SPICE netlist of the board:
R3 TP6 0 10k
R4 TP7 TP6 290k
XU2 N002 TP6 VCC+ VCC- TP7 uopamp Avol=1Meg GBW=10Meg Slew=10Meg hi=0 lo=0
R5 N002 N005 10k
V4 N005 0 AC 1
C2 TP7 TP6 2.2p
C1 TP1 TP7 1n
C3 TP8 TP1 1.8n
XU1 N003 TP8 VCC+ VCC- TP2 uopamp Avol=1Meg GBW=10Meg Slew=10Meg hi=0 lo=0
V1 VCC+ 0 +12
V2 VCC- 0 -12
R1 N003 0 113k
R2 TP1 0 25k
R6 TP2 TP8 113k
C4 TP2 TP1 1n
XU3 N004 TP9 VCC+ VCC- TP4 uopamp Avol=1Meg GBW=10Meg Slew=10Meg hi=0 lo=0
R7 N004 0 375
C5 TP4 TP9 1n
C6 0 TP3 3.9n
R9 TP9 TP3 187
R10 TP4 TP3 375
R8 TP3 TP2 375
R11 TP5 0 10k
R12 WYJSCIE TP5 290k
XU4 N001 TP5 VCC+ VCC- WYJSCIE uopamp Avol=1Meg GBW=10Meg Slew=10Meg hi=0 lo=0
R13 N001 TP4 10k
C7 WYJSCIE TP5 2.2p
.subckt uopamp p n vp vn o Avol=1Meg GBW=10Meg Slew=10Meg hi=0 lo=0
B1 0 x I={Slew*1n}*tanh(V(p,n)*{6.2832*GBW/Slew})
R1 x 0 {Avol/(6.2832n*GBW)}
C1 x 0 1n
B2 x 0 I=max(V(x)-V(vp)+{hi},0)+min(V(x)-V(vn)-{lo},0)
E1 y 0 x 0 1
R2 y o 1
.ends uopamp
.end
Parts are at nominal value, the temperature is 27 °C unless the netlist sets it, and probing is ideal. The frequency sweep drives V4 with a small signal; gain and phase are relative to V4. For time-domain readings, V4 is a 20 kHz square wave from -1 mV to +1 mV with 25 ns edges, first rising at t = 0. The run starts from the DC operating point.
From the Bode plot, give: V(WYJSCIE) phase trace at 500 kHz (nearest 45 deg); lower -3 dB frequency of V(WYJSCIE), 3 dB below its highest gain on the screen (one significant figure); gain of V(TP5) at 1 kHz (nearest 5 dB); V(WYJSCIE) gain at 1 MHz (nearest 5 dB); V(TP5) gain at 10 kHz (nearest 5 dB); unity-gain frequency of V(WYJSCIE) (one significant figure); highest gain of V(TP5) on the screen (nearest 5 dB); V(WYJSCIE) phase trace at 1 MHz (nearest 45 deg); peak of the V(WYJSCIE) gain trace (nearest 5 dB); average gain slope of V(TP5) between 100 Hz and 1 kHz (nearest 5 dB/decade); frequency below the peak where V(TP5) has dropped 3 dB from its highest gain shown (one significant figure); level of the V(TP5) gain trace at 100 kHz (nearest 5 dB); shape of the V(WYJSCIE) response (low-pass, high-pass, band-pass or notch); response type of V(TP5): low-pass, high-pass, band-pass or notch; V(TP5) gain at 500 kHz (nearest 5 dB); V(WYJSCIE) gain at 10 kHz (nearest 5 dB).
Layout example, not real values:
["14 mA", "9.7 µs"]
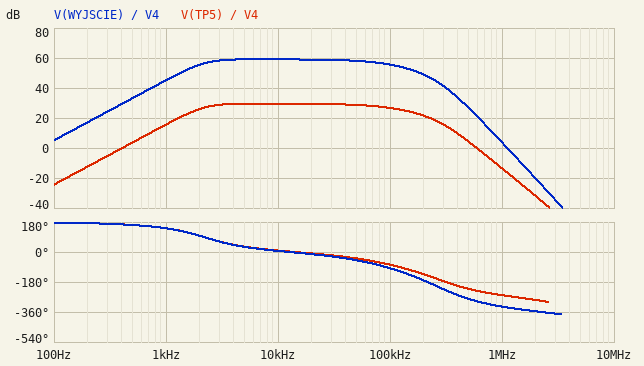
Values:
["-270 deg", "2 kHz", "15 dB", "5 dB", "30 dB", "1 MHz", "30 dB", "-315 deg", "60 dB", "40 dB/decade", "2 kHz", "25 dB", "band-pass", "band-pass", "5 dB", "60 dB"]
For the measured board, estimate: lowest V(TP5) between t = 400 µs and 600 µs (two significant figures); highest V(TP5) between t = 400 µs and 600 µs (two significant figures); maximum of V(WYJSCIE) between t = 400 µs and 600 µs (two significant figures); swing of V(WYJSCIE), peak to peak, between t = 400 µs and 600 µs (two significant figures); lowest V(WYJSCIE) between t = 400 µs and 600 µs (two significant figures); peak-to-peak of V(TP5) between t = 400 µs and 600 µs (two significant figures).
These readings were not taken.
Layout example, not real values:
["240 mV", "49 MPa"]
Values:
["-33 mV", "34 mV", "1.0 V", "2.0 V", "-1.0 V", "67 mV"]
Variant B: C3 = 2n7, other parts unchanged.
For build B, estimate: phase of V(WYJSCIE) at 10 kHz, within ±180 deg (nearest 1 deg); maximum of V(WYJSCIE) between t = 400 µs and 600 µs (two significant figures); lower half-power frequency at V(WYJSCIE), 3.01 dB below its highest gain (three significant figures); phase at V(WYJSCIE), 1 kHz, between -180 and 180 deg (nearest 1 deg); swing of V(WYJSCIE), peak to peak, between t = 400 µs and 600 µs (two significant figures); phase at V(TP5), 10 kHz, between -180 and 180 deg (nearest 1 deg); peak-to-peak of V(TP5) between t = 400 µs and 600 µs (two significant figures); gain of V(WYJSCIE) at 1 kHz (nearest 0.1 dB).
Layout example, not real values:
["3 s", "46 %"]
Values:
["3 deg", "990 mV", "1.74 kHz", "132 deg", "2.0 V", "6 deg", "66 mV", "48.5 dB"]
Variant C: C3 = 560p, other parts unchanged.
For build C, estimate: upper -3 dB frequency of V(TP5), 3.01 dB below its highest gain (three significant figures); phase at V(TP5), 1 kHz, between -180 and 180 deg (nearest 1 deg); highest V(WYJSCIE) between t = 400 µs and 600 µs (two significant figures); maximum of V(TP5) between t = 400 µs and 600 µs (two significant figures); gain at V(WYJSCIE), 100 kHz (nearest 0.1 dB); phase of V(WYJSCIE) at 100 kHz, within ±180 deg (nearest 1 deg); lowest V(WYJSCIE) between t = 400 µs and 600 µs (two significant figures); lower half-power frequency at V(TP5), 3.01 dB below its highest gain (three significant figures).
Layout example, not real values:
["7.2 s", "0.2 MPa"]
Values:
["109 kHz", "156 deg", "1.1 V", "38 mV", "55.6 dB", "-95 deg", "-1.1 V", "4.47 kHz"]
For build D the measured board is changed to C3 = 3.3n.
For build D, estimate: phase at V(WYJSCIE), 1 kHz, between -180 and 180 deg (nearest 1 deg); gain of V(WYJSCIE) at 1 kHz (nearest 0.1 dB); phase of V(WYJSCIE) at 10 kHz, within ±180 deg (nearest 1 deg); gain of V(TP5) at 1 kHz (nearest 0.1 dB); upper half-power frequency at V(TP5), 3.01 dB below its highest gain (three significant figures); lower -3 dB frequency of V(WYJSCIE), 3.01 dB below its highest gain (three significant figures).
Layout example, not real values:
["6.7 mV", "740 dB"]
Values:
["126 deg", "50.0 dB", "2 deg", "20.5 dB", "104 kHz", "1.60 kHz"]
